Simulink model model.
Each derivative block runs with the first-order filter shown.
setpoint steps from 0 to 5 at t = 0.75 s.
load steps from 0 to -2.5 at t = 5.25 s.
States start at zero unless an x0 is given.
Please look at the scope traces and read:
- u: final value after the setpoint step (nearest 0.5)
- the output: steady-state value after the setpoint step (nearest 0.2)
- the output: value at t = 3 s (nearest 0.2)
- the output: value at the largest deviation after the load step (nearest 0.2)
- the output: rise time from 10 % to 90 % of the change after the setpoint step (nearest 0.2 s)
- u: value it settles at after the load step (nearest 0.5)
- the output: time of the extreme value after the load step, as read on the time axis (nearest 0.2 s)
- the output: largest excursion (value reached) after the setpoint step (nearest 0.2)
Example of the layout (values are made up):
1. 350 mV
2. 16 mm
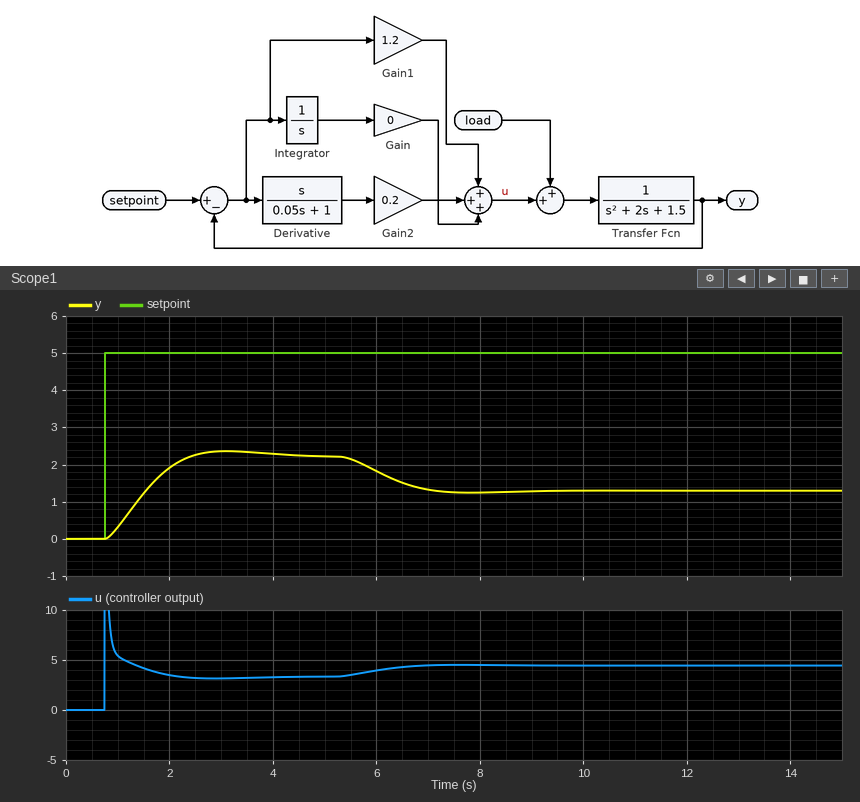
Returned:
1. 3.5
2. 2.2
3. 2.4
4. 1.2
5. 1.2 s
6. 4.5
7. 7.8 s
8. 2.4
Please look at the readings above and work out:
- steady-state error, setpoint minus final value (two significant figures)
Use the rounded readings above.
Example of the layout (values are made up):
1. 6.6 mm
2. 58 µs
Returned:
1. 2.8
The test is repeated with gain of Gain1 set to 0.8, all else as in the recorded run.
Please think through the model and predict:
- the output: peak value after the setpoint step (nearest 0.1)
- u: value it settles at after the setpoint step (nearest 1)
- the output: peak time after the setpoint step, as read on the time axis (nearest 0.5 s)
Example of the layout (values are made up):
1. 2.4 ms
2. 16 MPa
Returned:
1. 1.8
2. 3
3. 3.5 s
